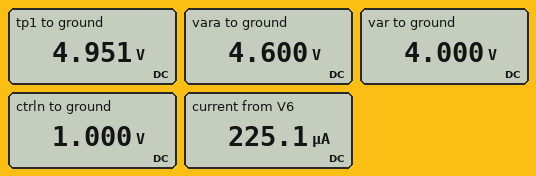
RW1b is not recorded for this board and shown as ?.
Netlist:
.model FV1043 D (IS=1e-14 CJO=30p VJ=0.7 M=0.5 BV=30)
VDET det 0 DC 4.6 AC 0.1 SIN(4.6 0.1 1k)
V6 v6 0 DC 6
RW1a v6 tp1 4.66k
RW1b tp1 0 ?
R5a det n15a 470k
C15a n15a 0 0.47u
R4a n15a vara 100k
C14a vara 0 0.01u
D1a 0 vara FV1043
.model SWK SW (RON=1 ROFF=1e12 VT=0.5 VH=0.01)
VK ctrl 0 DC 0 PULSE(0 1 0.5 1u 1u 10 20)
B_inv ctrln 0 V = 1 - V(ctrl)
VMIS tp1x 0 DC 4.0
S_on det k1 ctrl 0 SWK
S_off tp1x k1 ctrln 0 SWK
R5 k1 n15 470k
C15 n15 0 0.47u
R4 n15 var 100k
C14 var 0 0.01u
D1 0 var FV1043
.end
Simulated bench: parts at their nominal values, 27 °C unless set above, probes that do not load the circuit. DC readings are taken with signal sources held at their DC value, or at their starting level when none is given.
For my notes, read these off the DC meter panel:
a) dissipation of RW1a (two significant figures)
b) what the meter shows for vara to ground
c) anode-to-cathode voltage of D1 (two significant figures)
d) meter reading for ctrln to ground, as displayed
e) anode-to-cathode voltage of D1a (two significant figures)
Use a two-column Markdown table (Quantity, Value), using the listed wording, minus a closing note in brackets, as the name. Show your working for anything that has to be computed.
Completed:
| Quantity | Value |
|---|---|
| dissipation of RW1a | (6 V - 4.951 V)^2 / 4.66 kΩ = 240 µW |
| what the meter shows for vara to ground | 4.600 V |
| anode-to-cathode voltage of D1 | 0 V - 4 V = -4.0 V |
| meter reading for ctrln to ground, as displayed | 1.000 V |
| anode-to-cathode voltage of D1a | 0 V - 4.6 V = -4.6 V |
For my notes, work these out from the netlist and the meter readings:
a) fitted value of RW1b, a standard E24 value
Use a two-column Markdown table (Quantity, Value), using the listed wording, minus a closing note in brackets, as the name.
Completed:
| Quantity | Value |
|---|---|
| fitted value of RW1b, a standard E24 value | 22 kΩ |
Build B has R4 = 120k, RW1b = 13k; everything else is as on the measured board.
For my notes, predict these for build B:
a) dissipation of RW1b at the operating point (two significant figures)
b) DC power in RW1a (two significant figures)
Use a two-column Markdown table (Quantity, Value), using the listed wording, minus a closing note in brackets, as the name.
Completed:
| Quantity | Value |
|---|---|
| dissipation of RW1b at the operating point | 1.5 mW |
| DC power in RW1a | 540 µW |
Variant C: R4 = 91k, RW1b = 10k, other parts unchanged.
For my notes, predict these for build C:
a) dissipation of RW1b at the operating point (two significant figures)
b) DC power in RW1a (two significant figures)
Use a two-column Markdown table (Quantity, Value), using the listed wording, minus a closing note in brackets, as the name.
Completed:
| Quantity | Value |
|---|---|
| dissipation of RW1b at the operating point | 1.7 mW |
| DC power in RW1a | 780 µW |
